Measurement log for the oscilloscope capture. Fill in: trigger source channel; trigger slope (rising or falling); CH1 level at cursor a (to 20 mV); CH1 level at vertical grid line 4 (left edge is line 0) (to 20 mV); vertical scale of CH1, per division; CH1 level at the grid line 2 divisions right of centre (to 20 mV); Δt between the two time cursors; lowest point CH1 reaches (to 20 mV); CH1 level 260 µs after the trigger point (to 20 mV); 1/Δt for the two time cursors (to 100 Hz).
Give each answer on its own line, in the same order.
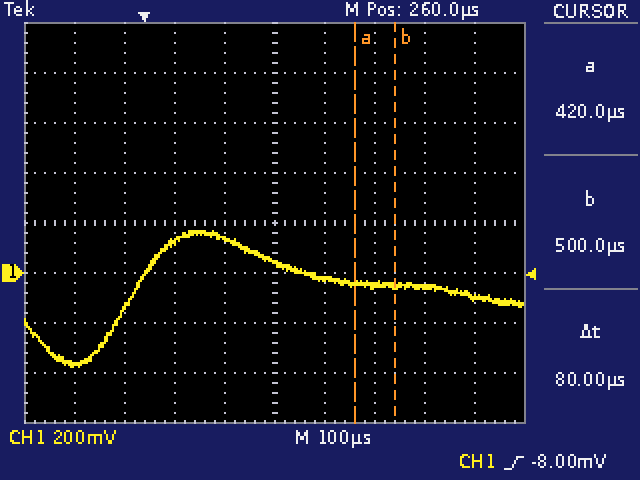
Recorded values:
CH1
rising
-40 mV
140 mV
200 mV
-60 mV
80 µs
-380 mV
40 mV
12.5 kHz
